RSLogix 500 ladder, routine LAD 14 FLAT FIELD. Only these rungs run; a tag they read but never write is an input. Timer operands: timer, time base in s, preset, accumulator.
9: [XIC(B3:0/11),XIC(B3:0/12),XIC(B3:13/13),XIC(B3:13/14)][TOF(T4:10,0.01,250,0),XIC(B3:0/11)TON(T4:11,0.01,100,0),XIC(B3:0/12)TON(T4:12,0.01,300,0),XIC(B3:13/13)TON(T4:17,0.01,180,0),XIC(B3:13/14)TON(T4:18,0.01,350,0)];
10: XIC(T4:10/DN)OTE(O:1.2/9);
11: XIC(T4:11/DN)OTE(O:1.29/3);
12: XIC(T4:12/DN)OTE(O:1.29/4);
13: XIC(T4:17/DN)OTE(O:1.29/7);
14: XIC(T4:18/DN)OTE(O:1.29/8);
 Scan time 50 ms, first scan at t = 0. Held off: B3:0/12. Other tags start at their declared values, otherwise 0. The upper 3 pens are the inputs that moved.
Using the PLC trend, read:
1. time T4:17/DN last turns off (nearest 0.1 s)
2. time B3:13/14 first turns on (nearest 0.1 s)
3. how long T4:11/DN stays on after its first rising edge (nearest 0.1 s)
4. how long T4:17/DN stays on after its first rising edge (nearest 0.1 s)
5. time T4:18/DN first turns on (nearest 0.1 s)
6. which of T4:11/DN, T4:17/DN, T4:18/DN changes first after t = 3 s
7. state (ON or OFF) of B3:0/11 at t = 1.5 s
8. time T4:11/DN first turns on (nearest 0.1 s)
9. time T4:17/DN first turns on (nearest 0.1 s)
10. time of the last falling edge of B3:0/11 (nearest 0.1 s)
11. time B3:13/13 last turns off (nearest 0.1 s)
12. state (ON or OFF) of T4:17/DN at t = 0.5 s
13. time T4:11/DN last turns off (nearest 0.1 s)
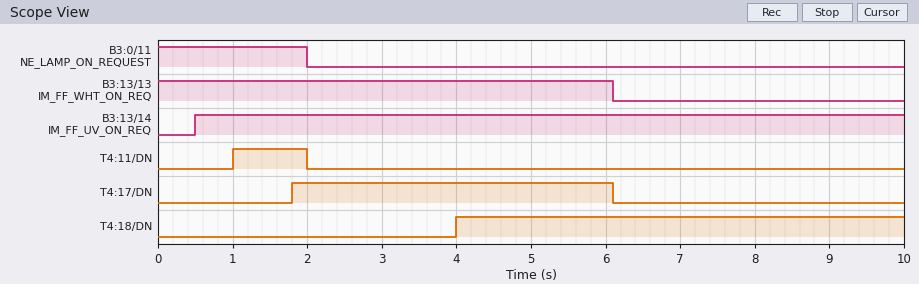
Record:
6.1 s
0.5 s
1.0 s
4.3 s
4.0 s
T4:18/DN
ON
1.0 s
1.8 s
2.0 s
6.1 s
OFF
2.0 s
